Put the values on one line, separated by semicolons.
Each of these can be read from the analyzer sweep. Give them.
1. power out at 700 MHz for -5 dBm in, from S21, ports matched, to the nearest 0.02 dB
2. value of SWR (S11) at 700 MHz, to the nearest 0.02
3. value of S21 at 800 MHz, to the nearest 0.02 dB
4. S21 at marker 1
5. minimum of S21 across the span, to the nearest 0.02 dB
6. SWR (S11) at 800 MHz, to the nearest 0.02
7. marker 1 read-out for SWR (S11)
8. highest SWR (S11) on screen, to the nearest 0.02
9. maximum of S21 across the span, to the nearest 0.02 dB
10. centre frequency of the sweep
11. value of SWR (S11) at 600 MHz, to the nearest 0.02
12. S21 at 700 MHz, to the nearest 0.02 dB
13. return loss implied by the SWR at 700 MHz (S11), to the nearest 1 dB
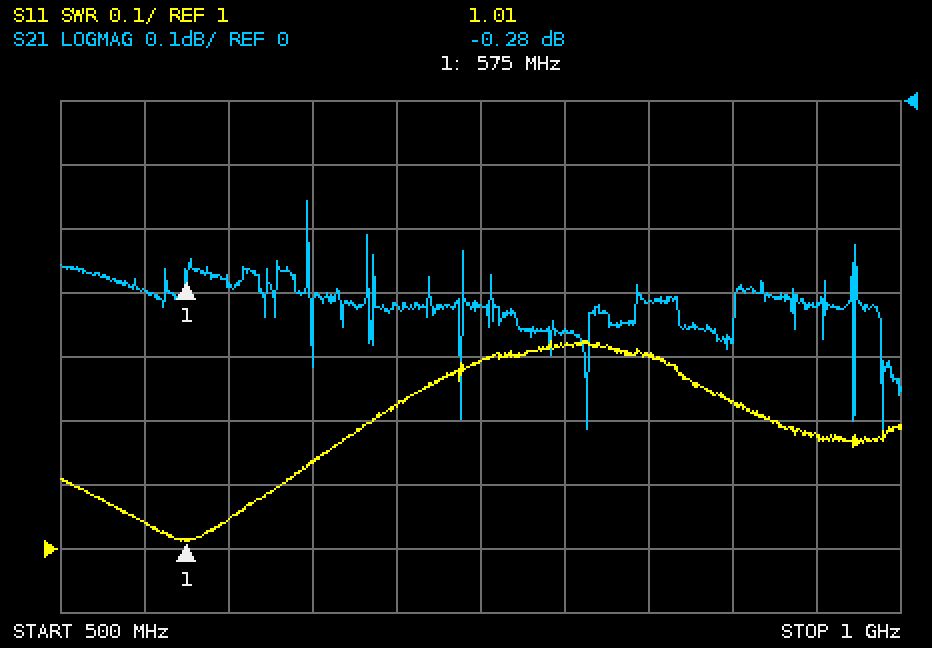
-5.32 dBm; 1.22; -0.36 dB; -0.28 dB; -0.52 dB; 1.32; 1.01; 1.32; -0.16 dB; 750 MHz; 1.04; -0.32 dB; 20 dB
